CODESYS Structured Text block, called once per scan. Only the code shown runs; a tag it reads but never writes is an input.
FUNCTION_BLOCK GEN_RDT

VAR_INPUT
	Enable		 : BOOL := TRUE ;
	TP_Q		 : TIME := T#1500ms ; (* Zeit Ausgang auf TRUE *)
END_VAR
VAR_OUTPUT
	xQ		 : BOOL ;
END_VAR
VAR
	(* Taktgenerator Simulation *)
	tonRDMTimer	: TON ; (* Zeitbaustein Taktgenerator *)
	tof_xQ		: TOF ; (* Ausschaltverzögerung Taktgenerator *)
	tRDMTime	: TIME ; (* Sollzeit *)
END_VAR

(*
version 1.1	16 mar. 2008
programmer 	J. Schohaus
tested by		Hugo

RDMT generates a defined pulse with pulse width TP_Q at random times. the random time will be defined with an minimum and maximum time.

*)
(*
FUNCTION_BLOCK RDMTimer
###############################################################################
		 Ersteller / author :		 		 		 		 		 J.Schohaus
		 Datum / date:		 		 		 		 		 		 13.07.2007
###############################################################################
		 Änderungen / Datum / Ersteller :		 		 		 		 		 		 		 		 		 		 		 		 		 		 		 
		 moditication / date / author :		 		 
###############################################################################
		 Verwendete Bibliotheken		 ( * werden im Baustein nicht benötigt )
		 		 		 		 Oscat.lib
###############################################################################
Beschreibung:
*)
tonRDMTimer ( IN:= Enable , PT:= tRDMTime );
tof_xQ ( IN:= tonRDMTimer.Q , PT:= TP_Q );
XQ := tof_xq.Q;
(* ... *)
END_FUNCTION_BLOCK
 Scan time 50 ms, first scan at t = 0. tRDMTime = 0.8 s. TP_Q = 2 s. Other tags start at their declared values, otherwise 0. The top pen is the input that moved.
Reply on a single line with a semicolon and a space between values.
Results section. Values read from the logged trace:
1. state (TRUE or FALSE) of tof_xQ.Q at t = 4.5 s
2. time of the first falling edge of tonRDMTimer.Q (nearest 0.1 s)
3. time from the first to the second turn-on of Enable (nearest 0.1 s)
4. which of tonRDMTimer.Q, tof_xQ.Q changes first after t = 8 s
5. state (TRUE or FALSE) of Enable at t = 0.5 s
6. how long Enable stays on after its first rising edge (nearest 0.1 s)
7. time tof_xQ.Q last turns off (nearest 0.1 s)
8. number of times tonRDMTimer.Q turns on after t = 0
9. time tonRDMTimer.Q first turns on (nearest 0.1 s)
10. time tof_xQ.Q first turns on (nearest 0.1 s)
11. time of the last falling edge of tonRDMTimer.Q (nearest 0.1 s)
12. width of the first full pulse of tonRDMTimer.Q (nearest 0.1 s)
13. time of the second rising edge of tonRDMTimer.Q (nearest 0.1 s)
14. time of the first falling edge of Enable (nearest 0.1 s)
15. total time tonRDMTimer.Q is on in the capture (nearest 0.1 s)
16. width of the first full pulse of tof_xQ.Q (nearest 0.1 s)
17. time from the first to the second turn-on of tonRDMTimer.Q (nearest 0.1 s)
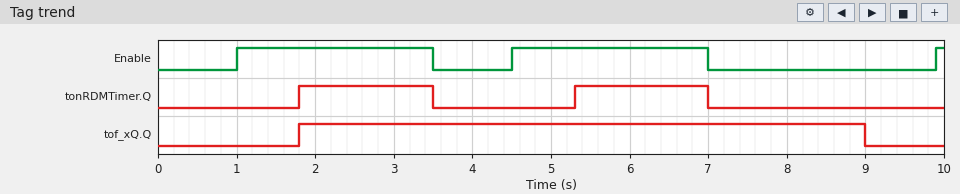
TRUE; 3.5 s; 3.5 s; tof_xQ.Q; FALSE; 2.5 s; 9.0 s; 2; 1.8 s; 1.8 s; 7.0 s; 1.7 s; 5.3 s; 3.5 s; 3.4 s; 7.2 s; 3.5 s
